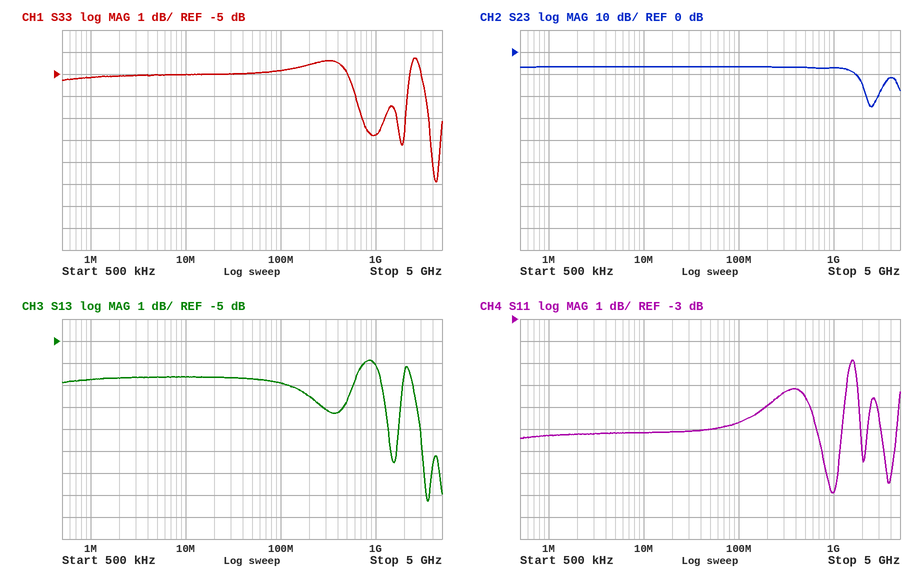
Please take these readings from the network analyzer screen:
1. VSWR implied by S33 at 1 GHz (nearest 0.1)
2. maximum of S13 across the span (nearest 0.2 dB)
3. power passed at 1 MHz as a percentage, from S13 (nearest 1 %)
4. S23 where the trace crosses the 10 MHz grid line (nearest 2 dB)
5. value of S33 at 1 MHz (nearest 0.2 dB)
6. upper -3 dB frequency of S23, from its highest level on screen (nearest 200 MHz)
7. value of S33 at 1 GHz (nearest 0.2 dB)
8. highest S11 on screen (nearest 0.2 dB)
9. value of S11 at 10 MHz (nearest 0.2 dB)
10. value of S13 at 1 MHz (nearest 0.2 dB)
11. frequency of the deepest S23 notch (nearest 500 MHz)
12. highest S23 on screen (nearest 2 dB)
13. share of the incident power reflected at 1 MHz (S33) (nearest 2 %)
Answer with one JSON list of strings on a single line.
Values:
["2.4", "-5.8 dB", "21 %", "-6 dB", "-5.2 dB", "1.6 GHz", "-7.8 dB", "-4.8 dB", "-8.2 dB", "-6.8 dB", "2.5 GHz", "-6 dB", "30 %"]
